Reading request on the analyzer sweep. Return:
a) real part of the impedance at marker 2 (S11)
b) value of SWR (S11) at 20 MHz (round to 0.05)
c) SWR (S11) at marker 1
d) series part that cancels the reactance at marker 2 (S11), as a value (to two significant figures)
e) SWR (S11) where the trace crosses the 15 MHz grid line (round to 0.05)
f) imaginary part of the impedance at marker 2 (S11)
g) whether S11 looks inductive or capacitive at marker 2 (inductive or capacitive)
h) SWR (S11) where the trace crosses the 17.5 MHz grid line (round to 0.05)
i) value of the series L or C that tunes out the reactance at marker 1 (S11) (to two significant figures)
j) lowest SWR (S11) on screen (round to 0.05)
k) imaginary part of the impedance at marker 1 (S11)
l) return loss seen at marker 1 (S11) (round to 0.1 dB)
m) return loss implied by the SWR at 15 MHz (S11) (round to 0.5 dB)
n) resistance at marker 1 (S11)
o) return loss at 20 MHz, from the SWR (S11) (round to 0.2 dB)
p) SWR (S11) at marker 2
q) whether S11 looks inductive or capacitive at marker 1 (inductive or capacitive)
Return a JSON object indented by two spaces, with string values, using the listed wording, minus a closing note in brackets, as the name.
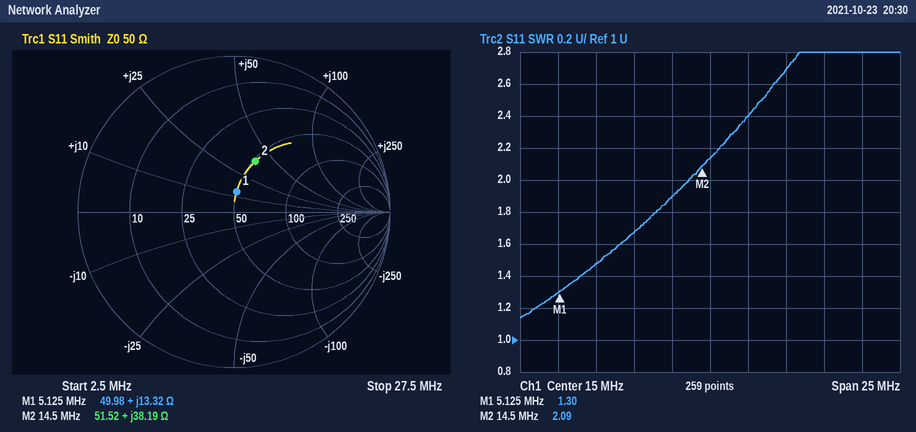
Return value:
{
  "real part of the impedance at marker 2": "51.52 Ω",
  "value of SWR (S11) at 20 MHz": "2.70",
  "SWR (S11) at marker 1": "1.30",
  "series part that cancels the reactance at marker 2 (S11), as a value": "290 pF",
  "SWR (S11) where the trace crosses the 15 MHz grid line": "2.15",
  "imaginary part of the impedance at marker 2": "+38.19 Ω",
  "whether S11 looks inductive or capacitive at marker 2": "inductive",
  "SWR (S11) where the trace crosses the 17.5 MHz grid line": "2.40",
  "value of the series L or C that tunes out the reactance at marker 1 (S11)": "2.3 nF",
  "lowest SWR (S11) on screen": "1.15",
  "imaginary part of the impedance at marker 1": "+13.32 Ω",
  "return loss seen at marker 1 (S11)": "17.6 dB",
  "return loss implied by the SWR at 15 MHz (S11)": "9.0 dB",
  "resistance at marker 1": "49.98 Ω",
  "return loss at 20 MHz, from the SWR (S11)": "6.8 dB",
  "SWR (S11) at marker 2": "2.09",
  "whether S11 looks inductive or capacitive at marker 1": "inductive"
}
